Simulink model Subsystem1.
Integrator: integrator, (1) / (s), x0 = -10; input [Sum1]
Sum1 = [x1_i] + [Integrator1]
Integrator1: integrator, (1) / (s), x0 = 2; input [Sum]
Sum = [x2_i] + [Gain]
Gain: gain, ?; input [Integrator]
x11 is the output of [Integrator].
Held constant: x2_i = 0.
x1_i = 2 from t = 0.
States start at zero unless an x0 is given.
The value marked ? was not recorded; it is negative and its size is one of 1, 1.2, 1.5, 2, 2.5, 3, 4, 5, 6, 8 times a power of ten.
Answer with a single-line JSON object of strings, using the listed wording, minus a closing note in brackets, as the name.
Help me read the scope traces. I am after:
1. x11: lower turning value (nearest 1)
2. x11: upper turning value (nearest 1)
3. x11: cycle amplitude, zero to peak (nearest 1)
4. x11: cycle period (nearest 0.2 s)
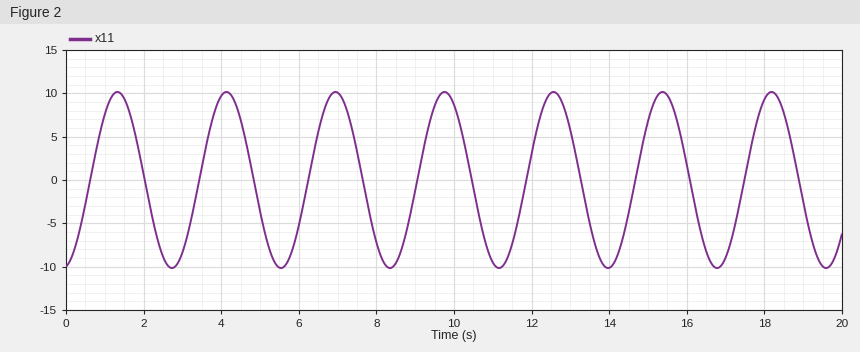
{"x11: lower turning value": "-10", "x11: upper turning value": "10", "x11: cycle amplitude, zero to peak": "10", "x11: cycle period": "2.8 s"}
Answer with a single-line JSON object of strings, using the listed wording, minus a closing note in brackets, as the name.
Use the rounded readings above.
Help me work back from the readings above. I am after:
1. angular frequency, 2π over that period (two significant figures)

{"angular frequency, 2π over that period": "2.2 rad/s"}
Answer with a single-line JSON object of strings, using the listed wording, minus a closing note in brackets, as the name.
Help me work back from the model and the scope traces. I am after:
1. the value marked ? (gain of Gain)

{"the value marked ?": "-5"}
